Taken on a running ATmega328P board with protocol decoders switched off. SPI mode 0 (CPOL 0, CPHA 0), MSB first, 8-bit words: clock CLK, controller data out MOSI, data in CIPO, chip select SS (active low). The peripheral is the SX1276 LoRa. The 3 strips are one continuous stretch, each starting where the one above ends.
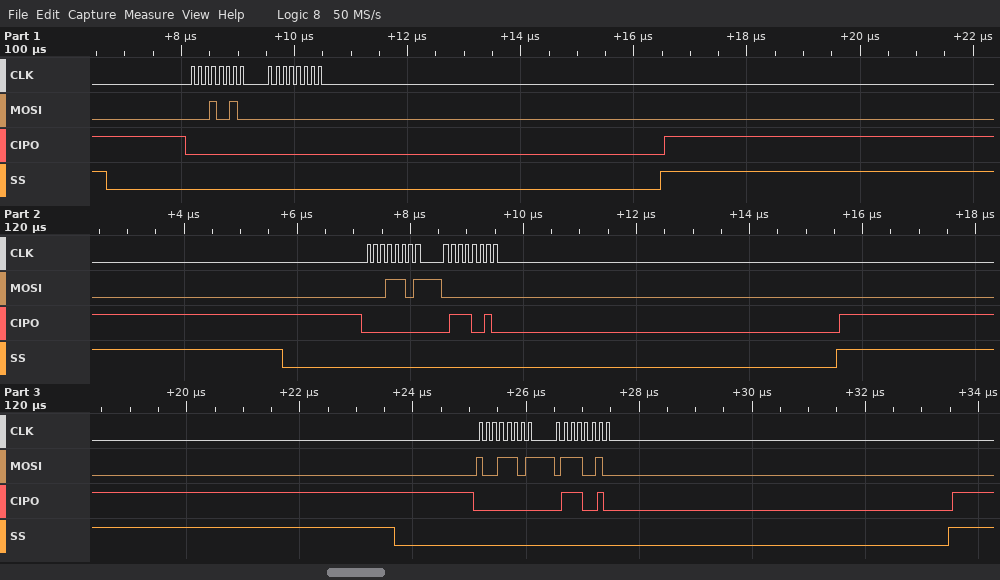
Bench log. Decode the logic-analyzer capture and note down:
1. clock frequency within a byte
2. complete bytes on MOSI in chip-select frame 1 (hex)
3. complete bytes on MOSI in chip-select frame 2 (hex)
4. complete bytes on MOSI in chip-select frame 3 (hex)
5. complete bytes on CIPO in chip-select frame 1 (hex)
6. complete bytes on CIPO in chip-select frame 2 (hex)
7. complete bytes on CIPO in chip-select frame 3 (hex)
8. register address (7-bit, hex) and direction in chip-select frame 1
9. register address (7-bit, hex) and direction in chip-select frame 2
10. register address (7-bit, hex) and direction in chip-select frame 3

8 MHz
12 00
1D 00
9D 72
00 00
00 72
00 72
0x12 read
0x1D read
0x1D write
